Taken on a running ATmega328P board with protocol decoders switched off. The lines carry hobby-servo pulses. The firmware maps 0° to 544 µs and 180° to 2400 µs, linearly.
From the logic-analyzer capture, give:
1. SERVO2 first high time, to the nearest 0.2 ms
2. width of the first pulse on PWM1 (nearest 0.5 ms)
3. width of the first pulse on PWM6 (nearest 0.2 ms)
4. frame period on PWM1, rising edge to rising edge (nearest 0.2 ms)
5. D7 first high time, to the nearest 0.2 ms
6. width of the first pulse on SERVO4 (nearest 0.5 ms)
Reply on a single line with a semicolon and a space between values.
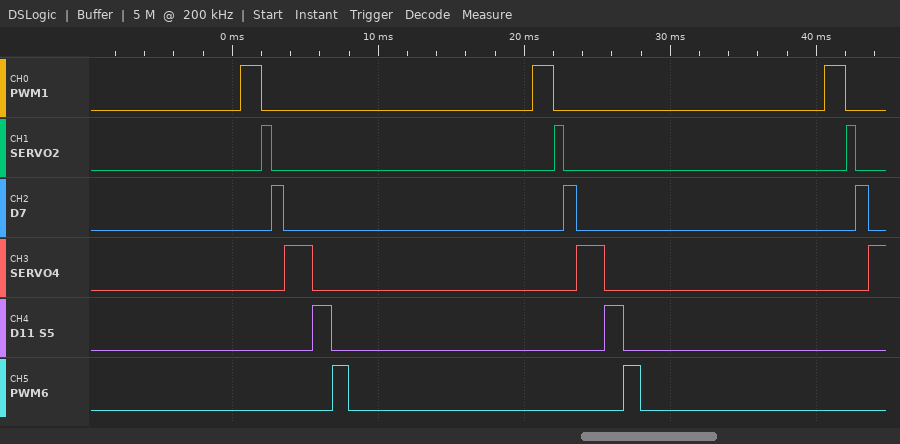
0.6 ms; 1.5 ms; 1.2 ms; 20.0 ms; 0.8 ms; 2.0 ms
